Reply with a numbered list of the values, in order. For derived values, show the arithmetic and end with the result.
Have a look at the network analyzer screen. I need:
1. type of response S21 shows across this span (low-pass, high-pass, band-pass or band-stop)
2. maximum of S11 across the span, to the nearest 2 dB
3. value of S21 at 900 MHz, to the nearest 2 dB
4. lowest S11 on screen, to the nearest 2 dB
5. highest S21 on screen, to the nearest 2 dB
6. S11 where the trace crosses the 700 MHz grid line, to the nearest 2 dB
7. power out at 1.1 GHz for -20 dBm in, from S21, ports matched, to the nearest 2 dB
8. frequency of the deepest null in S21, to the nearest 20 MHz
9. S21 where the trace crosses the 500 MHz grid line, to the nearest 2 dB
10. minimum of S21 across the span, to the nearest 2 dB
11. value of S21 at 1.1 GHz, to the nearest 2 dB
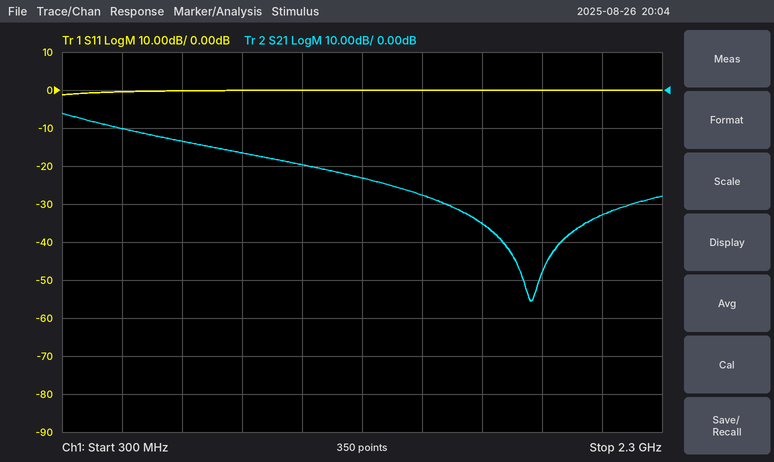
1. low-pass
2. 0 dB
3. -16 dB
4. -2 dB
5. -6 dB
6. 0 dB
7. -20 dBm + (-20 dB) = -40 dBm
8. 1.86 GHz
9. -10 dB
10. -56 dB
11. -20 dB
